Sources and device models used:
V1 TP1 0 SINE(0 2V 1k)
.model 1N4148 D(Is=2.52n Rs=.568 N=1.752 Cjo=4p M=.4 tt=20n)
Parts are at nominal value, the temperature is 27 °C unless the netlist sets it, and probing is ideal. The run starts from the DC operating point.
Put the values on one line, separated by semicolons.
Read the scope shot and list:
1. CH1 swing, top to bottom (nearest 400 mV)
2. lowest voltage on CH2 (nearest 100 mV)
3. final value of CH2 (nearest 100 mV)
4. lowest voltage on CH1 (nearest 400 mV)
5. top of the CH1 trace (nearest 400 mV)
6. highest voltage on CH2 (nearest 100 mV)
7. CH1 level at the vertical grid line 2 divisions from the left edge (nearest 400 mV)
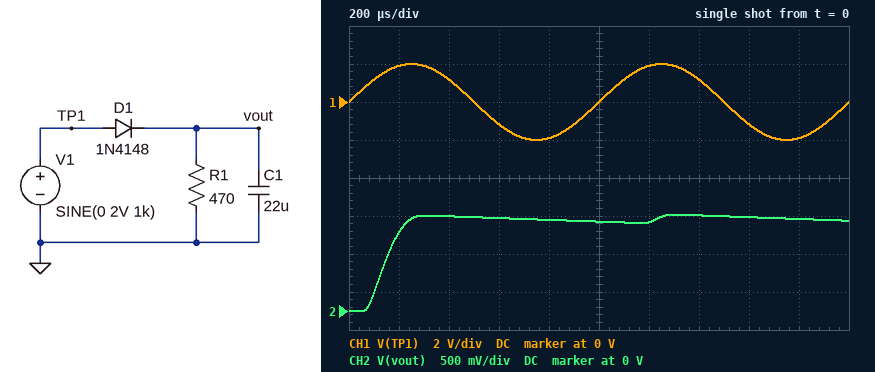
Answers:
4.0 V; 0 V; 1.2 V; -2.0 V; 2.0 V; 1.3 V; 1.2 V
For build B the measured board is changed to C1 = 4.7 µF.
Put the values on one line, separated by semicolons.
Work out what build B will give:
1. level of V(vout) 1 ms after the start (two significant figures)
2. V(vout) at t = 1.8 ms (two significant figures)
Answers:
970 mV; 1.1 V
